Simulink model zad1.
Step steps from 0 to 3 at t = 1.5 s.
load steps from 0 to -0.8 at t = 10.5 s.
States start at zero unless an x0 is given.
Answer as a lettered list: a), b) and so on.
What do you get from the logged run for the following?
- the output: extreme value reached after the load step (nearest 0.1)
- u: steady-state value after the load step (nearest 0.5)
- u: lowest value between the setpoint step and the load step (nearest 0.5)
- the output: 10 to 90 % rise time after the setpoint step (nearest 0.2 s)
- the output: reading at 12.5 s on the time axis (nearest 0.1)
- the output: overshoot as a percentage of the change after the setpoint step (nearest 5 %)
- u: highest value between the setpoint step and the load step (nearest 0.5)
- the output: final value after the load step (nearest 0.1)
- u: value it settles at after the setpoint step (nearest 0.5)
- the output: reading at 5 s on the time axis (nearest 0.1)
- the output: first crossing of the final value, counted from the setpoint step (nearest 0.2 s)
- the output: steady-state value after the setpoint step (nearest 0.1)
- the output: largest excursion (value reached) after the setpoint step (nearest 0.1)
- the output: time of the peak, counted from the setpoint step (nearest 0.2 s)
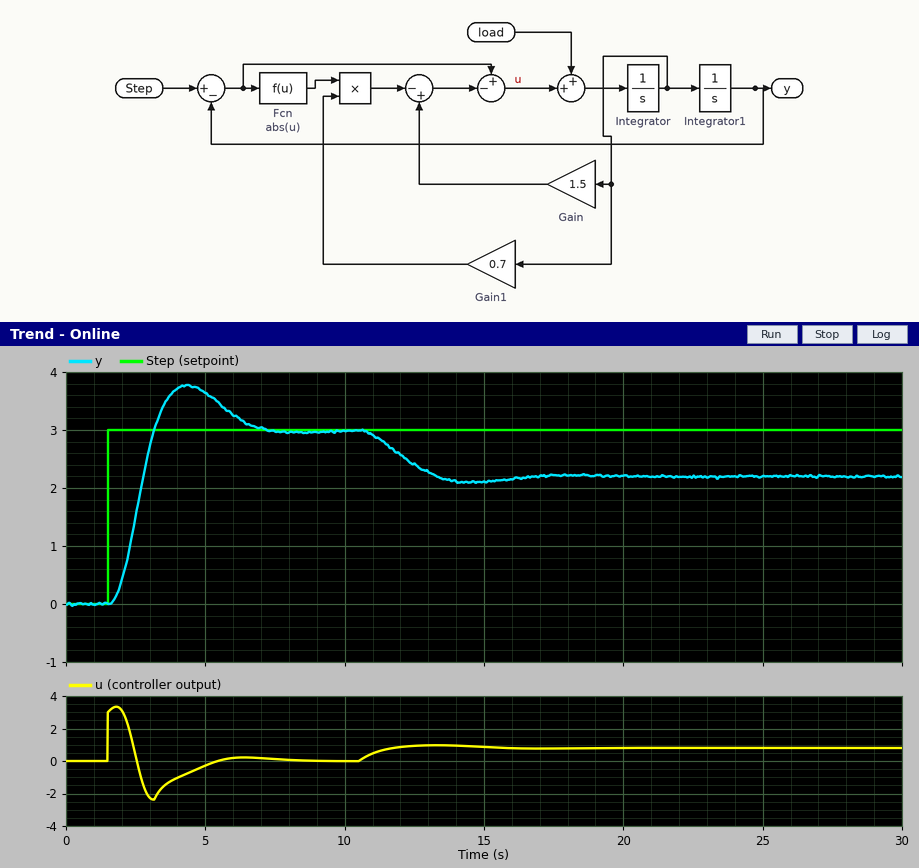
a) 2.1
b) 1.0
c) -2.5
d) 1.0 s
e) 2.4
f) 25 %
g) 3.5
h) 2.2
i) 0.0
j) 3.6
k) 1.6 s
l) 3.0
m) 3.8
n) 2.8 s
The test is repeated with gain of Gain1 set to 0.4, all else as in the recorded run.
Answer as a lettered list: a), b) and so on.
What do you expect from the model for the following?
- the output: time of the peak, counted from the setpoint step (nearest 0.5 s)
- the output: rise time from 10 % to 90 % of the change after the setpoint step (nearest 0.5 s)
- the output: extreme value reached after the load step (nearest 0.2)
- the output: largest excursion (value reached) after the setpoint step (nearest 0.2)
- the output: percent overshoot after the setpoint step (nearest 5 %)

a) 3.5 s
b) 1.5 s
c) 2.2
d) 3.4
e) 10 %
